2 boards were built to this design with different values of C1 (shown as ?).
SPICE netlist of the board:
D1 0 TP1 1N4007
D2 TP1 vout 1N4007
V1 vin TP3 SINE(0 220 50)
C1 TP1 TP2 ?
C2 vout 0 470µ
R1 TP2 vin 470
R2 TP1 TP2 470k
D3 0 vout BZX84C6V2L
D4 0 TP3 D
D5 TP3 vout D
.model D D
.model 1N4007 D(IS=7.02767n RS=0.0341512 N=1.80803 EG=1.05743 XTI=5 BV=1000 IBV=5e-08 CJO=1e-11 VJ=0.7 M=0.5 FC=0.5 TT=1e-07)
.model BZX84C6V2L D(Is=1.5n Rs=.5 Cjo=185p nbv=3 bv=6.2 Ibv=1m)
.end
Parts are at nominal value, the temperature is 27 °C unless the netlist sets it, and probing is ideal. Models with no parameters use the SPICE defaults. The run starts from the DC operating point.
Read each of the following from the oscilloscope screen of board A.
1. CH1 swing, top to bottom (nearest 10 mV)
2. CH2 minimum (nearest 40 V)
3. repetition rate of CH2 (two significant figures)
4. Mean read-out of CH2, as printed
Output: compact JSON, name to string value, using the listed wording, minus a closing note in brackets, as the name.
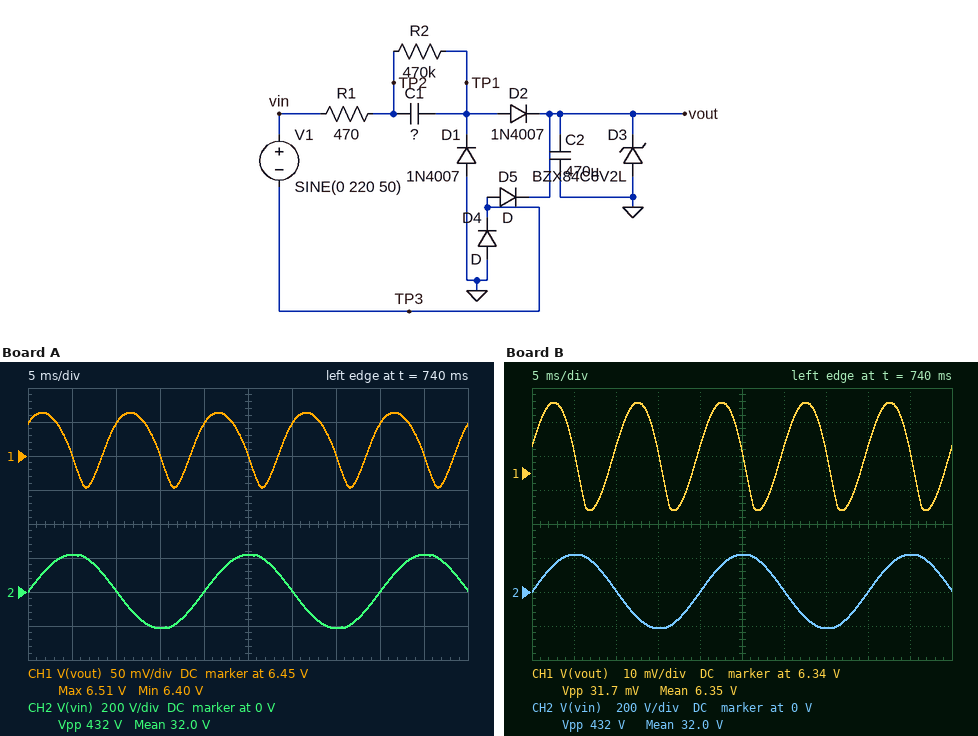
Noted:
{"CH1 swing, top to bottom": "110 mV", "CH2 minimum": "-200 V", "repetition rate of CH2": "50 Hz", "Mean read-out of CH2, as printed": "32.0 V"}
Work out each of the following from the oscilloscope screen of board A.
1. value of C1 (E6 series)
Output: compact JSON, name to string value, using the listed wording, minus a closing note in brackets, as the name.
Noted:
{"value of C1": "680 nF"}
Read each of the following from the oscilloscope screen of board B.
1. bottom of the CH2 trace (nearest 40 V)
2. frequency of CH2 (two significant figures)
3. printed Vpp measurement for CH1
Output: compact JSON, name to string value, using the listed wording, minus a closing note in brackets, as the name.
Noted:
{"bottom of the CH2 trace": "-200 V", "frequency of CH2": "50 Hz", "printed Vpp measurement for CH1": "31.7 mV"}
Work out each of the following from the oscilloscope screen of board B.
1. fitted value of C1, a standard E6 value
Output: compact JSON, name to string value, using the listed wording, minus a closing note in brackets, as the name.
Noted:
{"fitted value of C1, a standard E6 value": "150 nF"}
